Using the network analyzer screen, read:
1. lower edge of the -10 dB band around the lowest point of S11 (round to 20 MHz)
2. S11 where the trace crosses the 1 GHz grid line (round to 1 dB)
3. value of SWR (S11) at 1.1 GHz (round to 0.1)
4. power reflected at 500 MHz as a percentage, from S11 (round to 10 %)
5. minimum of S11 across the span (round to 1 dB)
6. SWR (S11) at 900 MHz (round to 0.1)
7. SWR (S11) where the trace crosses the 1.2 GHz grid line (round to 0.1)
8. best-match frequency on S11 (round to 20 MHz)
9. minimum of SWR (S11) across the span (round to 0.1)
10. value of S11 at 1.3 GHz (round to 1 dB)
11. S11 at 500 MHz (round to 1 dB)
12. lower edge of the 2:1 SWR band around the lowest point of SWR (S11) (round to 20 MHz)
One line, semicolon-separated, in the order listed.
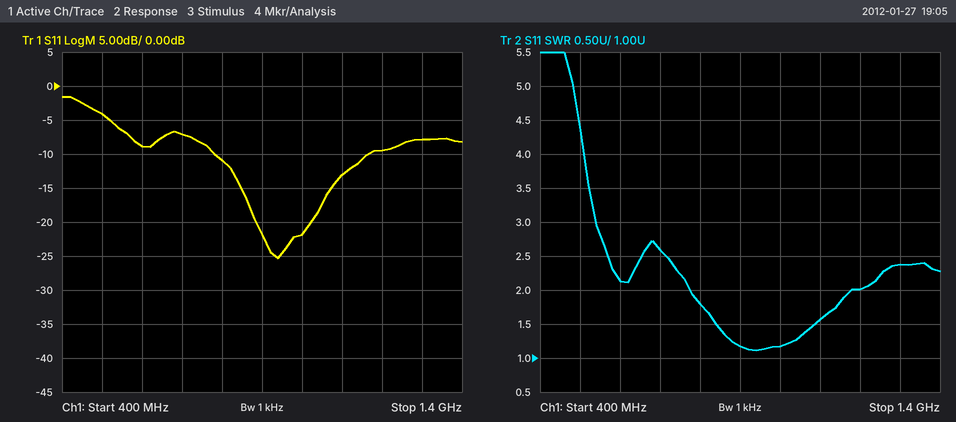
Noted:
780 MHz; -22 dB; 1.6; 40 %; -25 dB; 1.2; 2.0; 940 MHz; 1.1; -8 dB; -4 dB; 780 MHz
